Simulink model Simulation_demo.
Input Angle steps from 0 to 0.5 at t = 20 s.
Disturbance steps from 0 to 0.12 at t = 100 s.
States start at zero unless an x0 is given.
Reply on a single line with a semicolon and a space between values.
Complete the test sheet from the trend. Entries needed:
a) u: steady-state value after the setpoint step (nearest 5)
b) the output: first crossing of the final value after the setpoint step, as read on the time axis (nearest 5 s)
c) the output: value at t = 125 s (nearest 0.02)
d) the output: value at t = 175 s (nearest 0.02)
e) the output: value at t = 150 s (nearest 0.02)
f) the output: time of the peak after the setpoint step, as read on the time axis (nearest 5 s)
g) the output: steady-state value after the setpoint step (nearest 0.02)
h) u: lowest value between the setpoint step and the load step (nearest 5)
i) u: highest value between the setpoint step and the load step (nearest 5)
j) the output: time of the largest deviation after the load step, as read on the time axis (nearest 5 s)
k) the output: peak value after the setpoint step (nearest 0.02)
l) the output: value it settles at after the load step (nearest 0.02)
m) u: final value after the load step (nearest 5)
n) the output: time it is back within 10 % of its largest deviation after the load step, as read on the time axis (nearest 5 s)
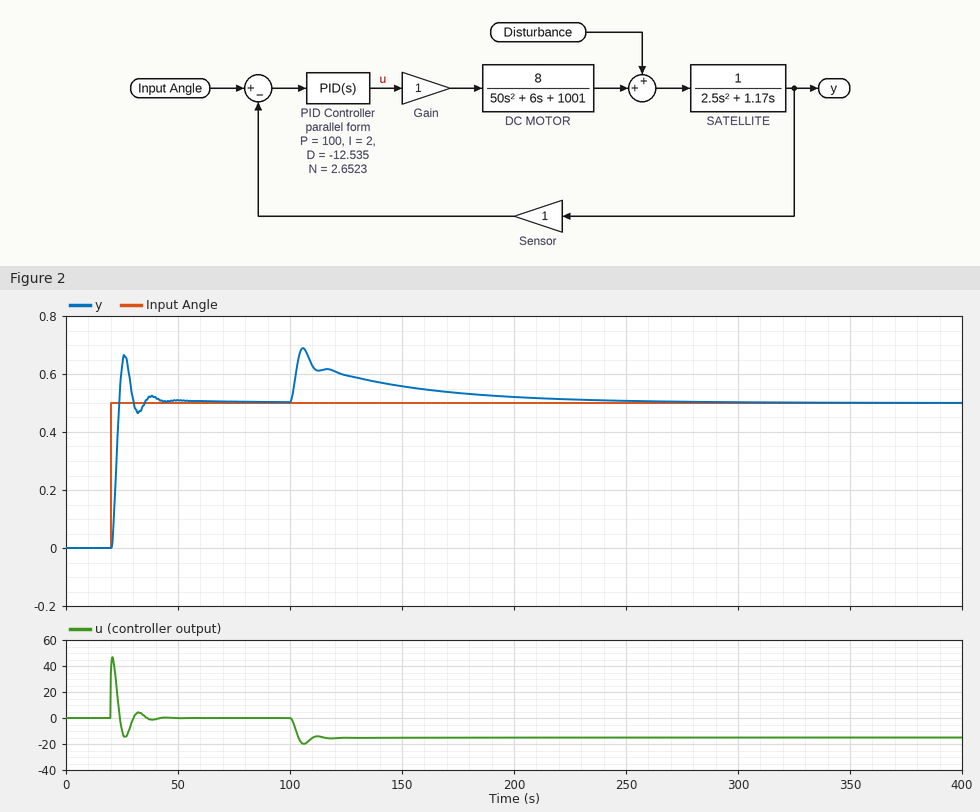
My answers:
0; 25 s; 0.60; 0.54; 0.56; 25 s; 0.50; -15; 45; 105 s; 0.66; 0.50; -15; 205 s
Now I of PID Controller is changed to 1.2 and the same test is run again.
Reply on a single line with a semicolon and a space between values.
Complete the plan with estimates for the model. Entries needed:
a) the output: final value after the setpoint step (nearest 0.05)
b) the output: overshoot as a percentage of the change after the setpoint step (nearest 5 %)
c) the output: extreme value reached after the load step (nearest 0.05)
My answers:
0.50; 30 %; 0.70
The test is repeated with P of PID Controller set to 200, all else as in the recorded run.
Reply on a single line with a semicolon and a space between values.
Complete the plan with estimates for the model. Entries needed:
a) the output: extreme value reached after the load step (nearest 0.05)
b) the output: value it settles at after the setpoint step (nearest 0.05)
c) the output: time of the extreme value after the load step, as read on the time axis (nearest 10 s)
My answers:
0.60; 0.50; 100 s
